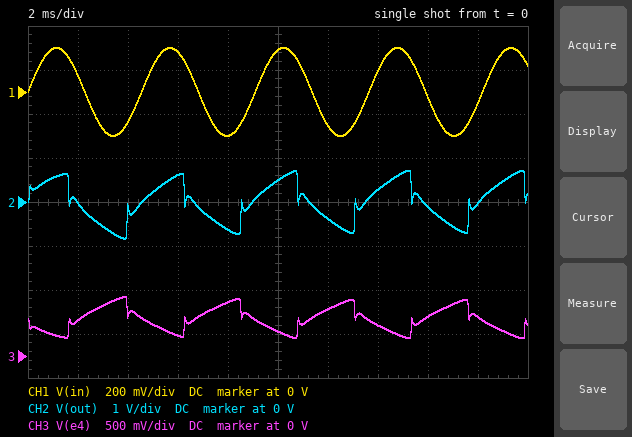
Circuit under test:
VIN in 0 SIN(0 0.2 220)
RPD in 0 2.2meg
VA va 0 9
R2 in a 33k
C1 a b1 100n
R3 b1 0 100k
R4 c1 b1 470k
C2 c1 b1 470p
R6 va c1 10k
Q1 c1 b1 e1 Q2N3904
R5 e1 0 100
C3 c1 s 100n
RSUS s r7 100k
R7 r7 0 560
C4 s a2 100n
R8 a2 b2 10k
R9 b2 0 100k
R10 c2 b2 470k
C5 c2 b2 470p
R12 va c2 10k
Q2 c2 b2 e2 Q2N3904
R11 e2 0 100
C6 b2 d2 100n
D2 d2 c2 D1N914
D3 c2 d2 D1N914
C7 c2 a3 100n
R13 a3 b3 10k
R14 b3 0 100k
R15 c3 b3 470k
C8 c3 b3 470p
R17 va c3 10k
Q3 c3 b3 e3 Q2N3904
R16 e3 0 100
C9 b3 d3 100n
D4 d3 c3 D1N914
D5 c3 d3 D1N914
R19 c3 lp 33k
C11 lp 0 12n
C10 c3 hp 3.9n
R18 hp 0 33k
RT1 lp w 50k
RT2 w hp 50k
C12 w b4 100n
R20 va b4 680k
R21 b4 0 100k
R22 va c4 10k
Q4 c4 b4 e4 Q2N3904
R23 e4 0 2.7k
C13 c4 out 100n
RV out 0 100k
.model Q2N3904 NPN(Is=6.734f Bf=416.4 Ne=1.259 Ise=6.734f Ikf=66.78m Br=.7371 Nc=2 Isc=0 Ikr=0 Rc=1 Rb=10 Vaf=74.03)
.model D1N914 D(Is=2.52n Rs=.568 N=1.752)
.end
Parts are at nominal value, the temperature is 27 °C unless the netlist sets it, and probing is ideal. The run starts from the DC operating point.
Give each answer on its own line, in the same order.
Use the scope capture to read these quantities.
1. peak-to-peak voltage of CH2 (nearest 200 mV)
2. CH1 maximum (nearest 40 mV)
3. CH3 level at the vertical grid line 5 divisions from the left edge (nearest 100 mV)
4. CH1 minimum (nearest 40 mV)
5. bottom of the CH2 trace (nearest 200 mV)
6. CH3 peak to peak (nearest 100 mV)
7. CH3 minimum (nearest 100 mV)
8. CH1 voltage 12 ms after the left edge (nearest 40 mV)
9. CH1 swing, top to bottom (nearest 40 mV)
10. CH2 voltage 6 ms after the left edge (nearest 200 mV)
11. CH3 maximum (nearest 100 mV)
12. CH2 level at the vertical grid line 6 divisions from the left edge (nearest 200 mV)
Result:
1.6 V
200 mV
300 mV
-200 mV
-800 mV
500 mV
200 mV
-160 mV
400 mV
600 mV
700 mV
-400 mV
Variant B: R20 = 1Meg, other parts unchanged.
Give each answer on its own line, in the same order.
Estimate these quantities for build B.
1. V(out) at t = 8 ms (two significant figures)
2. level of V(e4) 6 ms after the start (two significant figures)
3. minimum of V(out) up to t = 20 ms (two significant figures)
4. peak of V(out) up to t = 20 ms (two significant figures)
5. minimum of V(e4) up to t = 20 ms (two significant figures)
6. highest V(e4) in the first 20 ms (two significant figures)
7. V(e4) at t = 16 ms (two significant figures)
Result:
-600 mV
19 mV
-800 mV
540 mV
7.5 mV
410 mV
200 mV
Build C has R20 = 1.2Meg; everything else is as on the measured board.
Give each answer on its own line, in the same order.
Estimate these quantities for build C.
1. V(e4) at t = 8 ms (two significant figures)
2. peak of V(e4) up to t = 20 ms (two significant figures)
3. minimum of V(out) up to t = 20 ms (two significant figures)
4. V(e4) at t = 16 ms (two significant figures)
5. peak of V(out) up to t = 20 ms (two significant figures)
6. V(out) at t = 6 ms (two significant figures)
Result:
260 mV
320 mV
-750 mV
110 mV
340 mV
300 mV
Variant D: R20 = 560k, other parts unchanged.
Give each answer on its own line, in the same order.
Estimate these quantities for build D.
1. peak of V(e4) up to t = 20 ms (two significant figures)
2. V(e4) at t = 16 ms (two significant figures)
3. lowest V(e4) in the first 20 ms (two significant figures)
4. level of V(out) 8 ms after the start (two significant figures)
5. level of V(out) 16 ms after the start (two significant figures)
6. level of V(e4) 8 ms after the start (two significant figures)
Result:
840 mV
610 mV
360 mV
-640 mV
-130 mV
780 mV
